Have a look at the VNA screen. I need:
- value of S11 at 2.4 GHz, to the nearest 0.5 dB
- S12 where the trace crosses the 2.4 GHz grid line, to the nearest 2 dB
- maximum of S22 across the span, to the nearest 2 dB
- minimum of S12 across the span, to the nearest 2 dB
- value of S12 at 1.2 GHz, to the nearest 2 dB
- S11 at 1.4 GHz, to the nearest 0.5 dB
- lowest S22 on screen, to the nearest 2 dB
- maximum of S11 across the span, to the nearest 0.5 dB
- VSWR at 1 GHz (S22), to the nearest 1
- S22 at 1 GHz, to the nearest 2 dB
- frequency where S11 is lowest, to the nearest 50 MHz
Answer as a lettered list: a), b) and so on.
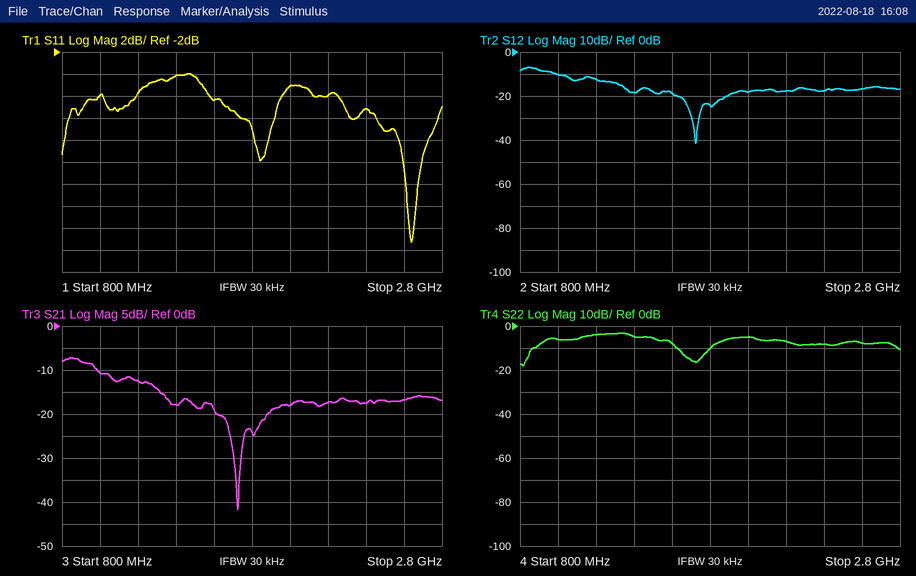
a) -7.0 dB
b) -18 dB
c) -4 dB
d) -42 dB
e) -12 dB
f) -4.0 dB
g) -18 dB
h) -4.0 dB
i) 3
j) -6 dB
k) 2.65 GHz
